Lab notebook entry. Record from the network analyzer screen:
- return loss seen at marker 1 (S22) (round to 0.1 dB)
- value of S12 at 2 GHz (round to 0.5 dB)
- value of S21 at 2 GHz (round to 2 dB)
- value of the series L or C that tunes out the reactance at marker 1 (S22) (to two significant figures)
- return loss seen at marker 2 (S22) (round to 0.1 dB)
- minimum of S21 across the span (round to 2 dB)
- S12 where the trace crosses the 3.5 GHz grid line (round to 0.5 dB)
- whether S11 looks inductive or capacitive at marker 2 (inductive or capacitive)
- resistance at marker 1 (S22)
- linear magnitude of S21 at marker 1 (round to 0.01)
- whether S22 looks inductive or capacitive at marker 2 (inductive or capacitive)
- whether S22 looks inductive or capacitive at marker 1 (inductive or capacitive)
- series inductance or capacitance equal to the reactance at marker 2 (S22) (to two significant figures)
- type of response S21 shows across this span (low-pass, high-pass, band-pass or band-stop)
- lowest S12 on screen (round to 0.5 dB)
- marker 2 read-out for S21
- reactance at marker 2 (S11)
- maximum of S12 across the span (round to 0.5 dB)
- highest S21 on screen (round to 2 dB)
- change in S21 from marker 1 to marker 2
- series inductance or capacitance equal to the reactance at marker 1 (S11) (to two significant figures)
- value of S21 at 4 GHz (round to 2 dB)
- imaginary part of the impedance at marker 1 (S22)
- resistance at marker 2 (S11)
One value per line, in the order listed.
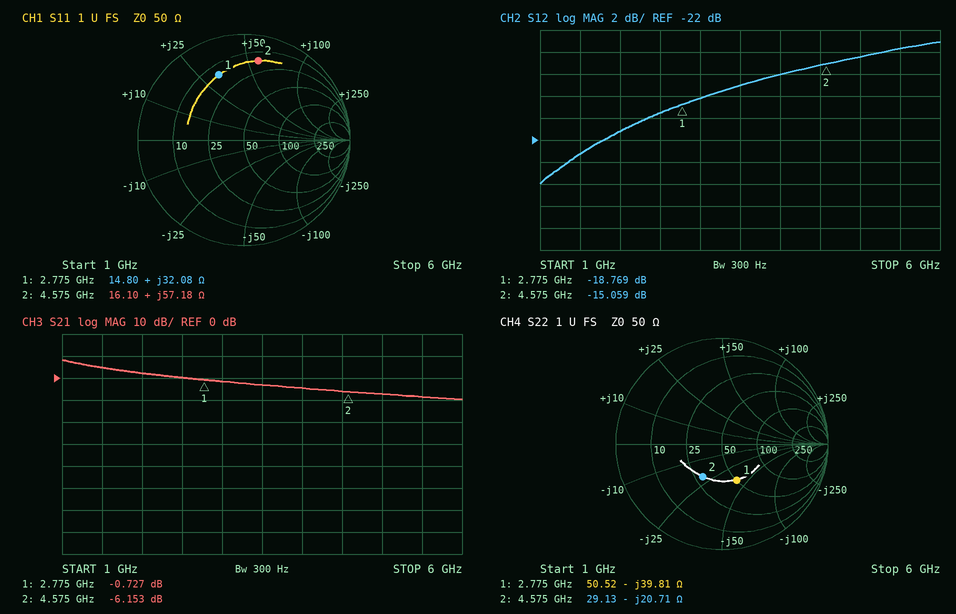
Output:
8.7 dB
-21.0 dB
2 dB
2.3 nH
8.9 dB
-10 dB
-17.0 dB
inductive
50.52 Ω
0.92
capacitive
capacitive
1.7 pF
low-pass
-26.0 dB
-6.153 dB
+57.18 Ω
-13.0 dB
8 dB
-5.426 dB
1.8 nH
-4 dB
-39.81 Ω
16.10 Ω
